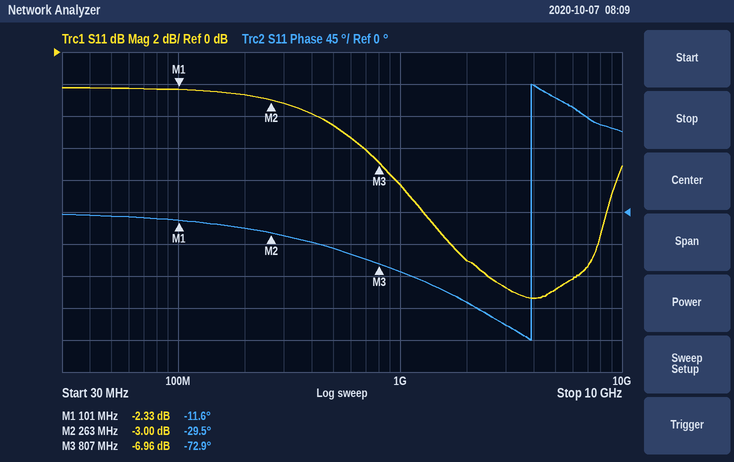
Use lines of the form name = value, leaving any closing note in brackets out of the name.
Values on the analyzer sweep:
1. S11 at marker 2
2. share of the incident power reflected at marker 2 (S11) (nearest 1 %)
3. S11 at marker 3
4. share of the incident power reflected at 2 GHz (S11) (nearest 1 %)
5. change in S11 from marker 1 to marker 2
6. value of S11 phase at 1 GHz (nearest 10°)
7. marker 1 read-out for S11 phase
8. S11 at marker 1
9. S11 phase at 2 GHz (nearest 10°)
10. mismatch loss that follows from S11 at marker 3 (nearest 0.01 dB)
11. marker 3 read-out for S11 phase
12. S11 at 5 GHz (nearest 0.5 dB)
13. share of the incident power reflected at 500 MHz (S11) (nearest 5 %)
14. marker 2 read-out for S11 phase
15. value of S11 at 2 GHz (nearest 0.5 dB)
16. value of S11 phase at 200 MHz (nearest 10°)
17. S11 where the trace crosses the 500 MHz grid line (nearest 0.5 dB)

S11 at marker 2 = -3.00 dB
share of the incident power reflected at marker 2 (S11) = 50 %
S11 at marker 3 = -6.96 dB
share of the incident power reflected at 2 GHz (S11) = 5 %
change in S11 from marker 1 to marker 2 = -0.67 dB
value of S11 phase at 1 GHz = -80°
marker 1 read-out for S11 phase = -11.6°
S11 at marker 1 = -2.33 dB
S11 phase at 2 GHz = -130°
mismatch loss that follows from S11 at marker 3 = 0.98 dB
marker 3 read-out for S11 phase = -72.9°
S11 at 5 GHz = -15.0 dB
share of the incident power reflected at 500 MHz (S11) = 35 %
marker 2 read-out for S11 phase = -29.5°
value of S11 at 2 GHz = -13.0 dB
value of S11 phase at 200 MHz = -20°
S11 where the trace crosses the 500 MHz grid line = -4.5 dB
